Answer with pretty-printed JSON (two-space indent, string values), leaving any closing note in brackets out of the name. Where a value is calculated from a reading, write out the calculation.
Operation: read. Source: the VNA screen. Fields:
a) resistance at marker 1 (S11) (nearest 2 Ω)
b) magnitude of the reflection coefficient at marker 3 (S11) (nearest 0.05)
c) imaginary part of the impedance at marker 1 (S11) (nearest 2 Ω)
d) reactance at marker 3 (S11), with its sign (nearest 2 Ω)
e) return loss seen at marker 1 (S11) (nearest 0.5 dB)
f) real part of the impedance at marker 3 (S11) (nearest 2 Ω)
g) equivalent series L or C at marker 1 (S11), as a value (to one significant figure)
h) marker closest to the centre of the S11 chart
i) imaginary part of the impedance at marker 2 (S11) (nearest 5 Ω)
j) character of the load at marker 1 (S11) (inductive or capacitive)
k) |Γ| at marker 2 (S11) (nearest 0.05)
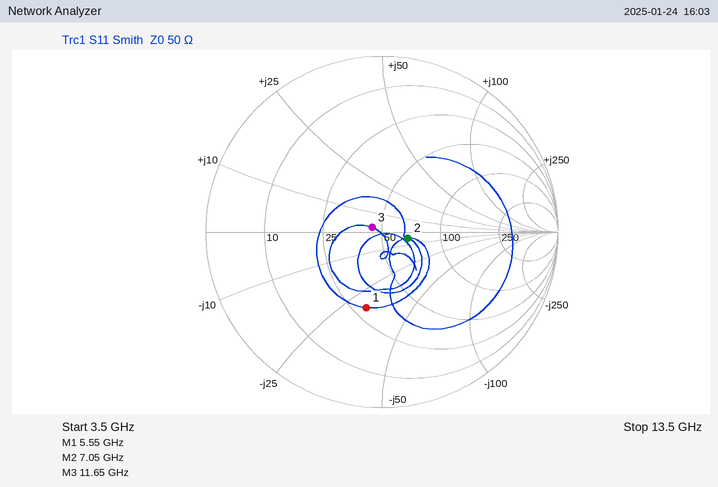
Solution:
{
  "resistance at marker 1 (S11)": "30 Ω",
  "magnitude of the reflection coefficient at marker 3 (S11)": "0.05",
  "imaginary part of the impedance at marker 1 (S11)": "-32 Ω",
  "reactance at marker 3 (S11), with its sign": "+2 Ω",
  "return loss seen at marker 1 (S11)": "7.0 dB",
  "real part of the impedance at marker 3 (S11)": "44 Ω",
  "equivalent series L or C at marker 1 (S11), as a value": "C = 1/(2π × 5.55 GHz × 32 Ω) ≈ 896 fF, so 900 fF to one significant figure",
  "marker closest to the centre of the S11 chart": "marker 3",
  "imaginary part of the impedance at marker 2 (S11)": "-5 Ω",
  "character of the load at marker 1 (S11)": "capacitive",
  "|Γ| at marker 2 (S11)": "0.15"
}
